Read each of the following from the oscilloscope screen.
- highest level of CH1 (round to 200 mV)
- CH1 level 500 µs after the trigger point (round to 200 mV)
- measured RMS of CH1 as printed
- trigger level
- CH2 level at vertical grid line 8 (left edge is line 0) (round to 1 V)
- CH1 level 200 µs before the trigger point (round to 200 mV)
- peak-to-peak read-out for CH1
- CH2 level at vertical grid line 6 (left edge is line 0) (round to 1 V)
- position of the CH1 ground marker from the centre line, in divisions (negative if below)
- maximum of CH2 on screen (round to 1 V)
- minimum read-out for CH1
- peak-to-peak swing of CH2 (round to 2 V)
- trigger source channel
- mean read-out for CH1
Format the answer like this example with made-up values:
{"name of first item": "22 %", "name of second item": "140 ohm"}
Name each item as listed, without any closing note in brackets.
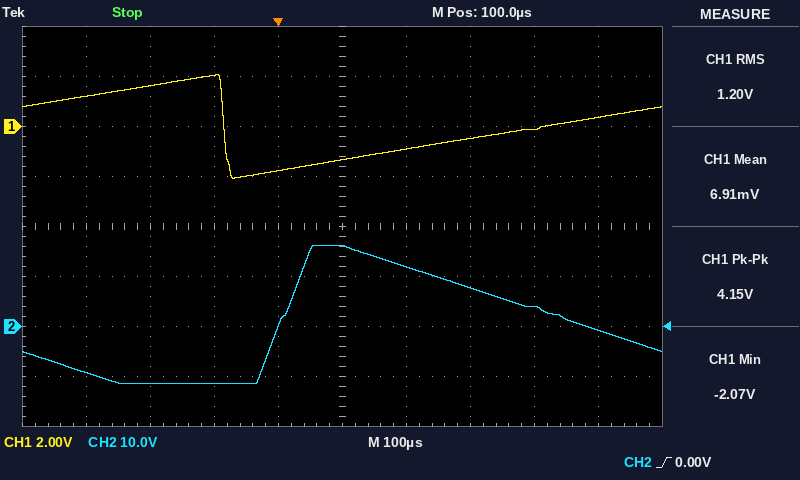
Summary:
{"highest level of CH1": "2.0 V", "CH1 level 500 µs after the trigger point": "400 mV", "measured RMS of CH1 as printed": "1.20 V", "trigger level": "0.00 V", "CH2 level at vertical grid line 8 (left edge is line 0)": "4 V", "CH1 level 200 µs before the trigger point": "1.6 V", "peak-to-peak read-out for CH1": "4.15 V", "CH2 level at vertical grid line 6 (left edge is line 0)": "12 V", "position of the CH1 ground marker from the centre line, in divisions": "+2.0 div", "maximum of CH2 on screen": "16 V", "minimum read-out for CH1": "-2.07 V", "peak-to-peak swing of CH2": "28 V", "trigger source channel": "CH2", "mean read-out for CH1": "6.91 mV"}
